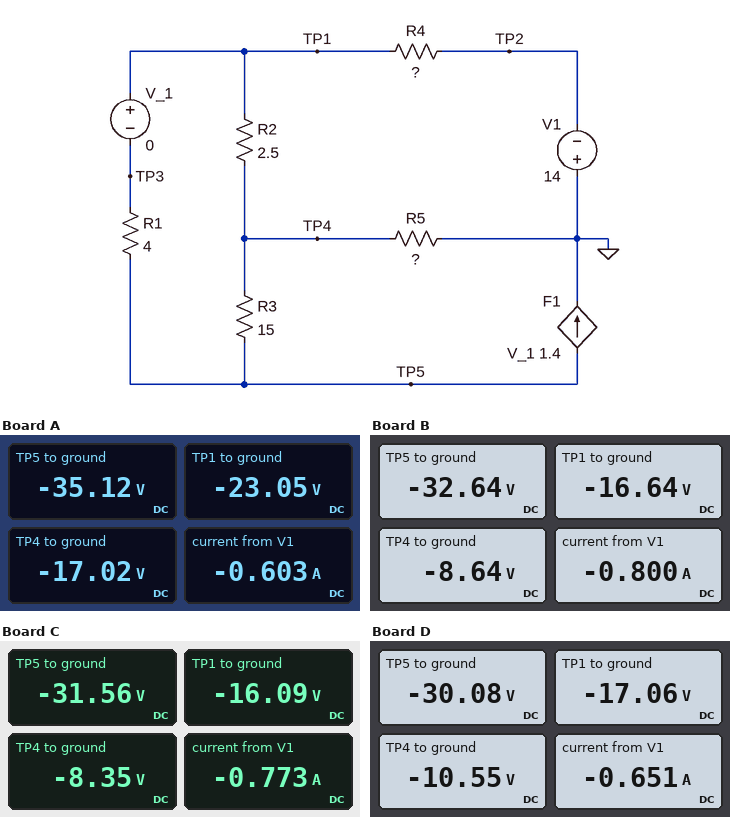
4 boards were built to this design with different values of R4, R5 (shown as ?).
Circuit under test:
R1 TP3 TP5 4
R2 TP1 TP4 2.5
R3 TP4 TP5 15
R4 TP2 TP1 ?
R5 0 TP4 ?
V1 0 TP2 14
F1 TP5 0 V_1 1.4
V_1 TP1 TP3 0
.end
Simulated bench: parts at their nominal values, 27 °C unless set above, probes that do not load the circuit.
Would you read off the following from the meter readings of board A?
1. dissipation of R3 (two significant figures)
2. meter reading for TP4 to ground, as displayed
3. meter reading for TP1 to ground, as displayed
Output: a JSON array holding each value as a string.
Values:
["22 W", "-17.02 V", "-23.05 V"]
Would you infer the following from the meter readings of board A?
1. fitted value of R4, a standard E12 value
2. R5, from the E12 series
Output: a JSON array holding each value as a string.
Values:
["15 Ω", "4.7 Ω"]
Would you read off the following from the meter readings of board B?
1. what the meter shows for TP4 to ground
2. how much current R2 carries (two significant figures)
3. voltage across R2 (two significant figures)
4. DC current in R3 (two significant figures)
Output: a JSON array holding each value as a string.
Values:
["-8.64 V", "3.2 A", "8.0 V", "1.6 A"]
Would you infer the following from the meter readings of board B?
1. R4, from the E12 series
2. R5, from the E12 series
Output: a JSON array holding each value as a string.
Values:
["3.3 Ω", "1.8 Ω"]
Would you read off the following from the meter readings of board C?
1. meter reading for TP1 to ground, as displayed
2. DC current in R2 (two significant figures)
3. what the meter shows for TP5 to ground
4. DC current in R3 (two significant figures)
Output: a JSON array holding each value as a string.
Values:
["-16.09 V", "3.1 A", "-31.56 V", "1.5 A"]
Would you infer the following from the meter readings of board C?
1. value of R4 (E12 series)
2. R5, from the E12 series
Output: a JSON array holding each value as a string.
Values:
["2.7 Ω", "1.8 Ω"]
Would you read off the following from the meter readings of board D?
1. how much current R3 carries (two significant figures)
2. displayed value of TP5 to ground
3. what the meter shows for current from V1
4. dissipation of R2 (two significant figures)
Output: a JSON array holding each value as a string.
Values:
["1.3 A", "-30.08 V", "-0.651 A", "17 W"]
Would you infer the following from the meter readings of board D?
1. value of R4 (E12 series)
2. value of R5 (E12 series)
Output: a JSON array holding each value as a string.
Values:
["4.7 Ω", "2.7 Ω"]
